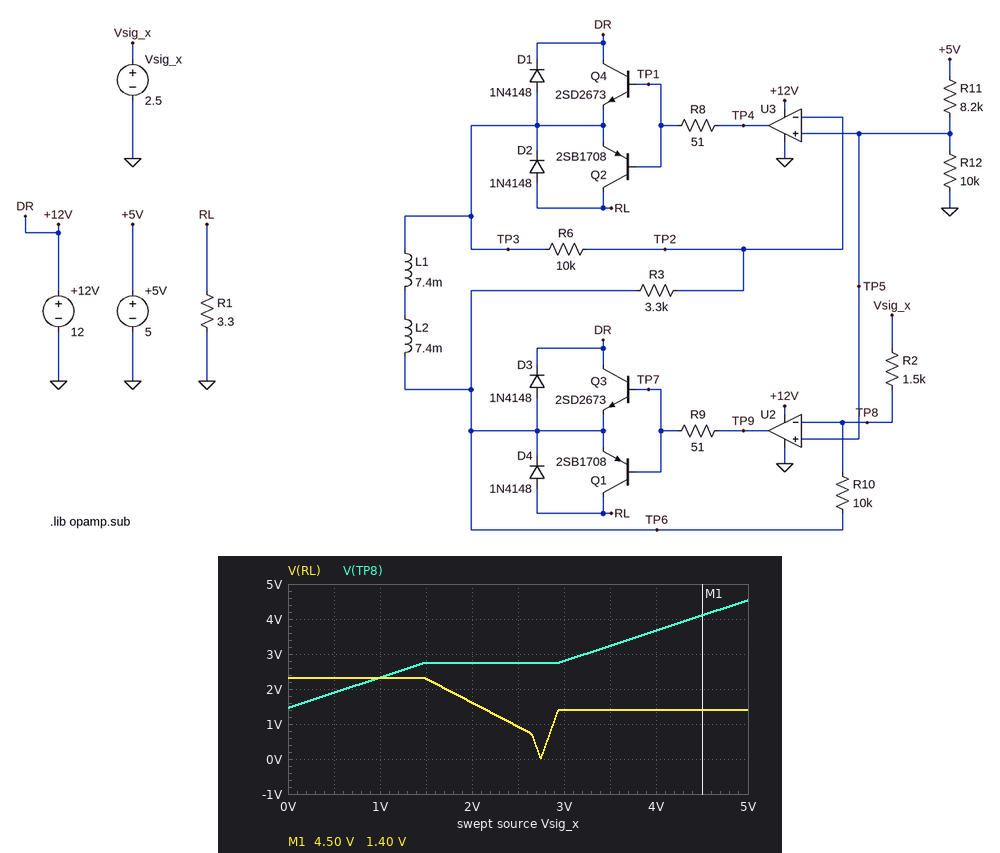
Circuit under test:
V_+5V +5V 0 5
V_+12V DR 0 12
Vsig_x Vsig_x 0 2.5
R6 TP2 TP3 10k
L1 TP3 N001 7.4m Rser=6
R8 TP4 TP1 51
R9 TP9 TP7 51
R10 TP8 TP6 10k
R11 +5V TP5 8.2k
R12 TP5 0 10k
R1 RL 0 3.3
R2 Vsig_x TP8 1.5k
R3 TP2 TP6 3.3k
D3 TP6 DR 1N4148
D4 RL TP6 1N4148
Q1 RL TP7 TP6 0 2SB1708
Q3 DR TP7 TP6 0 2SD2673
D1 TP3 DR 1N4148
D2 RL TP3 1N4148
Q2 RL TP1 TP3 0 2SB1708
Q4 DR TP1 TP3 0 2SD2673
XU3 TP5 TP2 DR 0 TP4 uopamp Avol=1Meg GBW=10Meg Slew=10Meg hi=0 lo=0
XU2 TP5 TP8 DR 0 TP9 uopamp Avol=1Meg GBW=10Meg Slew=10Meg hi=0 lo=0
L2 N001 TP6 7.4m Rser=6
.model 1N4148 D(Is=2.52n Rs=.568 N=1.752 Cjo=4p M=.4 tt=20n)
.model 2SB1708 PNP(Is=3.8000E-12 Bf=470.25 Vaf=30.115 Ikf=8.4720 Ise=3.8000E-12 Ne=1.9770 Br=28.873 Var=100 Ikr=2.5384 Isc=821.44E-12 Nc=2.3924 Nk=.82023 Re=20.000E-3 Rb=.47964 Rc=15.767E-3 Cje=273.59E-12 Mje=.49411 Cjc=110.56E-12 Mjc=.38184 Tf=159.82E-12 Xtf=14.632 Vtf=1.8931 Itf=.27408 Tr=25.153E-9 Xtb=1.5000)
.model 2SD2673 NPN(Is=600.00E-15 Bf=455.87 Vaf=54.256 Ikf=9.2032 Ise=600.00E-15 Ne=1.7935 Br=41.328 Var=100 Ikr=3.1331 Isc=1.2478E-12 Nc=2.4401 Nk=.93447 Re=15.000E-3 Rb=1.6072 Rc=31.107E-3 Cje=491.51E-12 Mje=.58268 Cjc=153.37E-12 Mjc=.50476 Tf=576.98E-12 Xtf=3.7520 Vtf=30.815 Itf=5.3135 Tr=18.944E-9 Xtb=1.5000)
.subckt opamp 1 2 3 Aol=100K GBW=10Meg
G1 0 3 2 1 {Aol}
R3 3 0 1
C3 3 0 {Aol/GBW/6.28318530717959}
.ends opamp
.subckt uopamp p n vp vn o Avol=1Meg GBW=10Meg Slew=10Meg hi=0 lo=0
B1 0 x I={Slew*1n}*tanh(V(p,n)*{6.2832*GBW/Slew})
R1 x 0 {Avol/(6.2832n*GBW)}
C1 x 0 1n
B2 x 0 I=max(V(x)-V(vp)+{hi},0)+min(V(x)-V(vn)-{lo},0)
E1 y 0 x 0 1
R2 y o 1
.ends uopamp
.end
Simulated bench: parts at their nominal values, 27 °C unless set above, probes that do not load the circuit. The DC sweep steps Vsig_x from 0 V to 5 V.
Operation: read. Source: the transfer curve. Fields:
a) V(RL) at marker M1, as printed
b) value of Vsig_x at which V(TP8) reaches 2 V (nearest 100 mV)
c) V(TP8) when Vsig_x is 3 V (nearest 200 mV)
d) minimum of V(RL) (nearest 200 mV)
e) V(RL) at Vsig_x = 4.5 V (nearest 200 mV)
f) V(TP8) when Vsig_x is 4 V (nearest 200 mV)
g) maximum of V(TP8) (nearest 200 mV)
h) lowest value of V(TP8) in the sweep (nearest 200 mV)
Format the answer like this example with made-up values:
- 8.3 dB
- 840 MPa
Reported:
- 1.40 V
- 600 mV
- 2.8 V
- 0 V
- 1.4 V
- 3.6 V
- 4.6 V
- 1.4 V
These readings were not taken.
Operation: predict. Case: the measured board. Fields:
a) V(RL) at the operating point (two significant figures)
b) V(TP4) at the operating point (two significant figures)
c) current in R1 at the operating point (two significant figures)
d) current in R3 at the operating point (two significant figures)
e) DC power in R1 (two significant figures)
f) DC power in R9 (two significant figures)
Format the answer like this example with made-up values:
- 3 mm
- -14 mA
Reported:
- 920 mV
- -4.1 mV
- 280 mA
- 260 µA
- 260 mW
- 18 µW
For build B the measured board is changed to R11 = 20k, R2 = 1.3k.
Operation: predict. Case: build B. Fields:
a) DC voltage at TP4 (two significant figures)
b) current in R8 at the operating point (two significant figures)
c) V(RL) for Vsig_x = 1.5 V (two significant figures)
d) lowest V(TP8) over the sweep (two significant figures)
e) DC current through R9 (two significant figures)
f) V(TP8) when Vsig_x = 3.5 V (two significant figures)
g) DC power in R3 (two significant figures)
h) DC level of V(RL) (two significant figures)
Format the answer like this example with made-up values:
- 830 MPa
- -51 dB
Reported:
- 4.7 V
- 530 µA
- 620 mV
- 1.3 V
- 4.5 mA
- 3.2 V
- 180 µW
- 850 mV
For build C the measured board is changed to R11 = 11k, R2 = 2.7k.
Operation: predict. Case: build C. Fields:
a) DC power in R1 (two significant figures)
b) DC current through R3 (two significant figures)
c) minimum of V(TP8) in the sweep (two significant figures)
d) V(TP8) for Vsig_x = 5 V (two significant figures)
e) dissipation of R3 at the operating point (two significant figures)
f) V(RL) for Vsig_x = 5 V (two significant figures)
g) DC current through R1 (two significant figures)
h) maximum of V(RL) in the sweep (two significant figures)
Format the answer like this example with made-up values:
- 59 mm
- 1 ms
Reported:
- 72 mW
- 130 µA
- 2.4 V
- 4.2 V
- 59 µW
- 1.2 V
- 150 mA
- 2.3 V
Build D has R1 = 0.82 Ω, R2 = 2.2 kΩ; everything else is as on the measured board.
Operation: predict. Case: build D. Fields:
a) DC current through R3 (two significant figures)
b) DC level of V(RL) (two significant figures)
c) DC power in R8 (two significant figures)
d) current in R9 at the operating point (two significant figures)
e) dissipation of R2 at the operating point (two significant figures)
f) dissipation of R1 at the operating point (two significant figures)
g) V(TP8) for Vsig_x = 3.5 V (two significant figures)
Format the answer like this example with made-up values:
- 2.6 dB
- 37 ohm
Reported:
- 240 µA
- 220 mV
- 19 µW
- 540 µA
- 28 µW
- 58 mW
- 3.0 V
